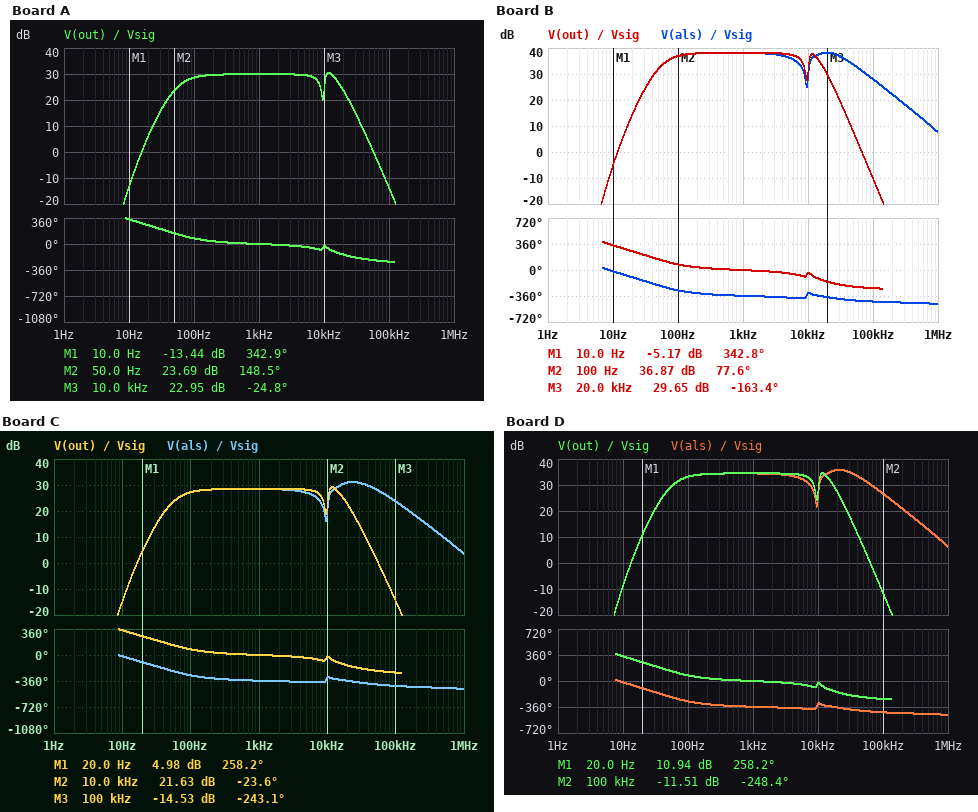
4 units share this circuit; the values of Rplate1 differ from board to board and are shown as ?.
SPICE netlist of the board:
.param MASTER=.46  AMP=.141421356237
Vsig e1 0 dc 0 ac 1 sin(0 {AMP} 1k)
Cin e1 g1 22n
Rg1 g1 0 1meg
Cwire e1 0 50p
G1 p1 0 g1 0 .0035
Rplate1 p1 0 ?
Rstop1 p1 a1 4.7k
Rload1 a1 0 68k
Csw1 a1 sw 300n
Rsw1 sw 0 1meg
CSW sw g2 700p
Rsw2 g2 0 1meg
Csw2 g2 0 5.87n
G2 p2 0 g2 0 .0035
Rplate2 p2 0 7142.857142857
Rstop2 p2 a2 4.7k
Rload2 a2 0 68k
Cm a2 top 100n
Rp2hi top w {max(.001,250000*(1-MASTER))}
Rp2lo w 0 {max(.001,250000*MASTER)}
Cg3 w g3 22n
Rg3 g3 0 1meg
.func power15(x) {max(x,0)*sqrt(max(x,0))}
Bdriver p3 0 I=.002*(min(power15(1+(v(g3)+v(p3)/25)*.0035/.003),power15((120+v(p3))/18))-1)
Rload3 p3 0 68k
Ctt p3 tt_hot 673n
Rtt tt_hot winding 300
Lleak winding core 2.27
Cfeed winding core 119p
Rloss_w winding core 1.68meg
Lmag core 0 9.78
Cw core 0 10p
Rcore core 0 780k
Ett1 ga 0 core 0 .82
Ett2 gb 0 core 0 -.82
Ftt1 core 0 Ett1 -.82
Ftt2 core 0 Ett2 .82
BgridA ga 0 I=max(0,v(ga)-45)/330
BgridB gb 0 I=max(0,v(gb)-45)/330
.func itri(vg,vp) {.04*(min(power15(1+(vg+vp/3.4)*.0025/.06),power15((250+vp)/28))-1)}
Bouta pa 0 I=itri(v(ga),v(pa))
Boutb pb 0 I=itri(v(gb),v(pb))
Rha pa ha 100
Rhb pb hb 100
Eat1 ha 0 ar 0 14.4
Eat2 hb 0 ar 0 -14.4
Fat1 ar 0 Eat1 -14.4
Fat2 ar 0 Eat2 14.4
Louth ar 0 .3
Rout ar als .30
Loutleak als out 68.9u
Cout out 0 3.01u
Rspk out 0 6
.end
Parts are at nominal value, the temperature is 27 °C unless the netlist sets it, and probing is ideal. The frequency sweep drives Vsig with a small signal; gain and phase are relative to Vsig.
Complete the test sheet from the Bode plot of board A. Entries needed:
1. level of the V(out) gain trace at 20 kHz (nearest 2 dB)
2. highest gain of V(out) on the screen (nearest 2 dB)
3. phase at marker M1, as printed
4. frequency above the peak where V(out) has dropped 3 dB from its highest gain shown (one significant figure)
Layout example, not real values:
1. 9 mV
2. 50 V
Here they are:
1. 24 dB
2. 30 dB
3. 342.9 deg
4. 20 kHz
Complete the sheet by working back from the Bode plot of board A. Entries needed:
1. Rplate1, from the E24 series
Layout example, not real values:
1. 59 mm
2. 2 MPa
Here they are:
1. 5.1 kΩ
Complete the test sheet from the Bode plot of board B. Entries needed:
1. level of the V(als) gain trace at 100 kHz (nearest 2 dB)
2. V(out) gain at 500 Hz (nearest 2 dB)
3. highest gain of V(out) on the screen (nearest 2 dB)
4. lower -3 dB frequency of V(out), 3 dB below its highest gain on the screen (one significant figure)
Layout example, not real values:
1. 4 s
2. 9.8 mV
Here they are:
1. 28 dB
2. 38 dB
3. 38 dB
4. 70 Hz
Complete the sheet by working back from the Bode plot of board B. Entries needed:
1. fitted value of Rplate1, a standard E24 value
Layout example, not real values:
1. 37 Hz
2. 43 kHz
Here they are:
1. 15 kΩ
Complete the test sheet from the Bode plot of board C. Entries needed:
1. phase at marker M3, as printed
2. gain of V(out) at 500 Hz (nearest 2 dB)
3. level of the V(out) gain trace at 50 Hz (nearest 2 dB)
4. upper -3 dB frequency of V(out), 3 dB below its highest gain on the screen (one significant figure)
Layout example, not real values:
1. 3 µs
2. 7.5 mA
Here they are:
1. -243.1 deg
2. 28 dB
3. 22 dB
4. 20 kHz
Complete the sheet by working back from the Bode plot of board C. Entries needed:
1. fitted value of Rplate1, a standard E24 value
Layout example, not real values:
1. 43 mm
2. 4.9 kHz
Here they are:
1. 4.3 kΩ
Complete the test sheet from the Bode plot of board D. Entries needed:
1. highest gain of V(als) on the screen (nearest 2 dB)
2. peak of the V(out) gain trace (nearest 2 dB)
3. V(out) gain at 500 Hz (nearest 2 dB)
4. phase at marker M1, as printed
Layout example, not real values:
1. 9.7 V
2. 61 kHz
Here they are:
1. 36 dB
2. 34 dB
3. 34 dB
4. 258.2 deg
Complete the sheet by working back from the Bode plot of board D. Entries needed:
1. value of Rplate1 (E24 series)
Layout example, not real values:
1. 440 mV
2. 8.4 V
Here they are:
1. 9.1 kΩ
